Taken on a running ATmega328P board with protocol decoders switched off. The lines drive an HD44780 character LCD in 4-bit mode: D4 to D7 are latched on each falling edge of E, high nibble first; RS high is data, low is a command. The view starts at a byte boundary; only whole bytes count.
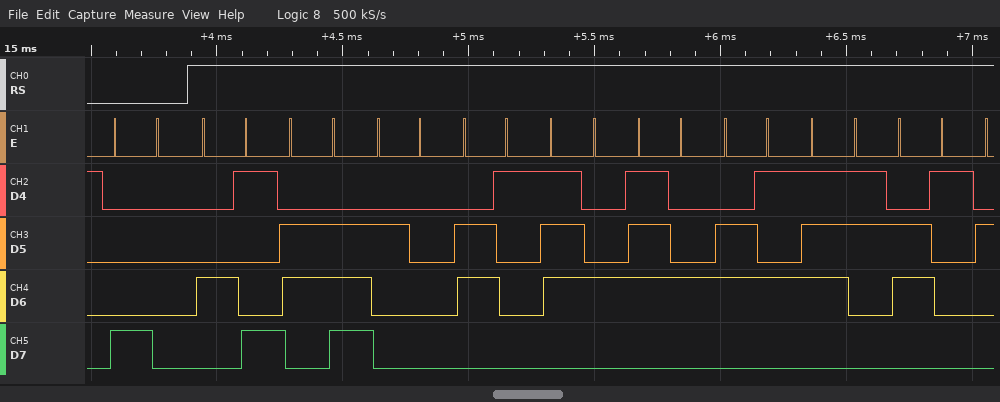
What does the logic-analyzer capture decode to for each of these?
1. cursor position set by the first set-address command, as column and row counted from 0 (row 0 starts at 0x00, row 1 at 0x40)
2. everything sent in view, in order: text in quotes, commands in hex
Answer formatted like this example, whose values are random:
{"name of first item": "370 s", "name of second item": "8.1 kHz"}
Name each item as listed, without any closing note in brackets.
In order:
{"cursor position set by the first set-address command, as column and row counted from 0": "column 0, row 0", "everything sent in view, in order: text in quotes, commands in hex": "0x80 \"In attesa\""}
